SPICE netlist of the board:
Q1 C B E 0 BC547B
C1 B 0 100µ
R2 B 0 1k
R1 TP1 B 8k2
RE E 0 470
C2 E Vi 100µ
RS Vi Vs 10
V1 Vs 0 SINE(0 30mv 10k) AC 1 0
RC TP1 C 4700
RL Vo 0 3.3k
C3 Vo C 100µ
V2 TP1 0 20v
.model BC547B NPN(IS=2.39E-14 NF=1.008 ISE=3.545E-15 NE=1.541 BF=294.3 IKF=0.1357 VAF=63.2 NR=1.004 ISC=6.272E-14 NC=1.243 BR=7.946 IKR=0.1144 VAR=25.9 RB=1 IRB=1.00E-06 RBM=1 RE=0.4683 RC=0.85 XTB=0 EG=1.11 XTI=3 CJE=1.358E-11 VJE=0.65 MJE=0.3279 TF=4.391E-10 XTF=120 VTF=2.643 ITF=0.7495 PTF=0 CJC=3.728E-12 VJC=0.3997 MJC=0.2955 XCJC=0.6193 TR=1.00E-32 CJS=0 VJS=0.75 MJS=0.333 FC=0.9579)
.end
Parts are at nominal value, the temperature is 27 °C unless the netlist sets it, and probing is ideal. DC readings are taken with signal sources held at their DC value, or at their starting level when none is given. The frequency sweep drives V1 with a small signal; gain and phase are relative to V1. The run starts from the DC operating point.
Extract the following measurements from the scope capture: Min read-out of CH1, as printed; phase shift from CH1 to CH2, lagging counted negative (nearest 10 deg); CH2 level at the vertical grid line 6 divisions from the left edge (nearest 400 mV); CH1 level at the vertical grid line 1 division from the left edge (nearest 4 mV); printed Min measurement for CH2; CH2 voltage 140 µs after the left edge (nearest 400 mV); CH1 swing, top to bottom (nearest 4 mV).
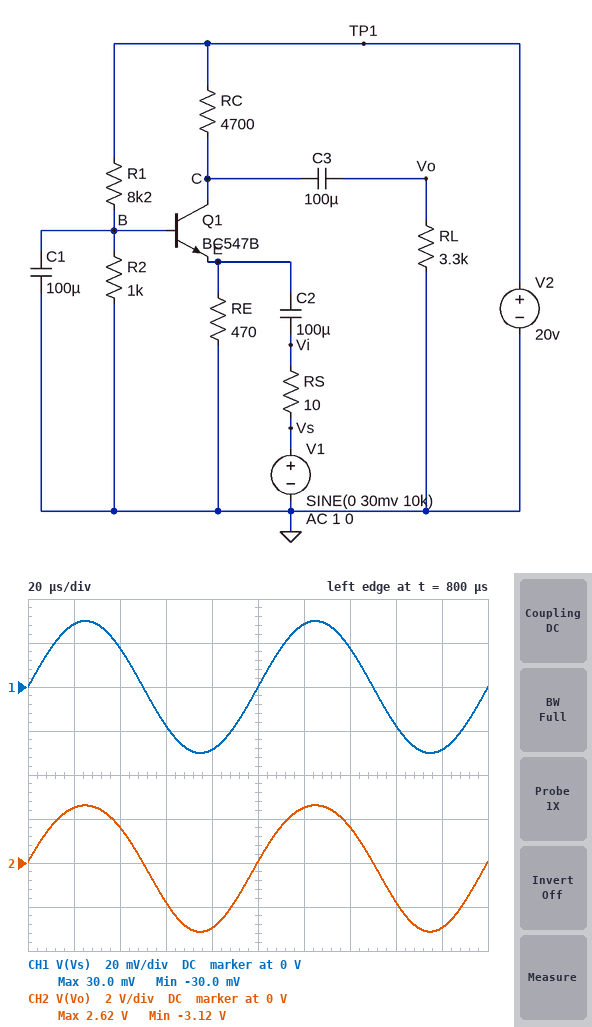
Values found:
-30.0 mV
0 deg
2.4 V
28 mV
-3.12 V
1.6 V
60 mV
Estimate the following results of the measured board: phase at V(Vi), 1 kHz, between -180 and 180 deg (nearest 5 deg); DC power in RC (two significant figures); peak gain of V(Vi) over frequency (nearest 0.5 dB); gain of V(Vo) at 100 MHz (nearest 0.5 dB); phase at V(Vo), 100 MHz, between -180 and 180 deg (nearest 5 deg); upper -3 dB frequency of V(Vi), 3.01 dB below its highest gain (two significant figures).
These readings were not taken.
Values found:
-5 deg
47 mW
0 dB
31.0 dB
-85 deg
110 Hz
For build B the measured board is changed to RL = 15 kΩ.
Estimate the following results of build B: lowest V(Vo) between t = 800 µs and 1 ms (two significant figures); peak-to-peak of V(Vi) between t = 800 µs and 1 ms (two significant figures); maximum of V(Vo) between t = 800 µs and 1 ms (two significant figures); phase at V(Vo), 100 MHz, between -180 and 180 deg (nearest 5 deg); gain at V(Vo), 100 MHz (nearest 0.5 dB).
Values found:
-3.6 V
34 mV
4.7 V
-95 deg
31.5 dB
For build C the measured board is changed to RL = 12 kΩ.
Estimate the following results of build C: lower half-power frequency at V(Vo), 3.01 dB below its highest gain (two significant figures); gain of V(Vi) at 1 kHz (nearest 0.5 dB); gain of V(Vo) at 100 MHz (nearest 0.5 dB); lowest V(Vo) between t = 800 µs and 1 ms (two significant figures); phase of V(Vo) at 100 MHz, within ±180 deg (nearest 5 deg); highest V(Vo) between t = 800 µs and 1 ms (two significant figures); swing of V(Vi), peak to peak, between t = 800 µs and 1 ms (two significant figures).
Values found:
80 Hz
-6.0 dB
31.5 dB
-3.6 V
-95 deg
4.4 V
34 mV
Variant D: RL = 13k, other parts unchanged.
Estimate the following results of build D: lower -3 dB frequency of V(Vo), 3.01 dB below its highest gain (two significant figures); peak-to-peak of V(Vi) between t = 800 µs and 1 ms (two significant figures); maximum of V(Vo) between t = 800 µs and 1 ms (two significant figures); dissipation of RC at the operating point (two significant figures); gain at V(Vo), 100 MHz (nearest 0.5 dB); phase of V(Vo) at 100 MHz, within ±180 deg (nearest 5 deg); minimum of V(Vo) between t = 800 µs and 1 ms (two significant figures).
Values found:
80 Hz
34 mV
4.5 V
47 mW
31.5 dB
-95 deg
-3.6 V
